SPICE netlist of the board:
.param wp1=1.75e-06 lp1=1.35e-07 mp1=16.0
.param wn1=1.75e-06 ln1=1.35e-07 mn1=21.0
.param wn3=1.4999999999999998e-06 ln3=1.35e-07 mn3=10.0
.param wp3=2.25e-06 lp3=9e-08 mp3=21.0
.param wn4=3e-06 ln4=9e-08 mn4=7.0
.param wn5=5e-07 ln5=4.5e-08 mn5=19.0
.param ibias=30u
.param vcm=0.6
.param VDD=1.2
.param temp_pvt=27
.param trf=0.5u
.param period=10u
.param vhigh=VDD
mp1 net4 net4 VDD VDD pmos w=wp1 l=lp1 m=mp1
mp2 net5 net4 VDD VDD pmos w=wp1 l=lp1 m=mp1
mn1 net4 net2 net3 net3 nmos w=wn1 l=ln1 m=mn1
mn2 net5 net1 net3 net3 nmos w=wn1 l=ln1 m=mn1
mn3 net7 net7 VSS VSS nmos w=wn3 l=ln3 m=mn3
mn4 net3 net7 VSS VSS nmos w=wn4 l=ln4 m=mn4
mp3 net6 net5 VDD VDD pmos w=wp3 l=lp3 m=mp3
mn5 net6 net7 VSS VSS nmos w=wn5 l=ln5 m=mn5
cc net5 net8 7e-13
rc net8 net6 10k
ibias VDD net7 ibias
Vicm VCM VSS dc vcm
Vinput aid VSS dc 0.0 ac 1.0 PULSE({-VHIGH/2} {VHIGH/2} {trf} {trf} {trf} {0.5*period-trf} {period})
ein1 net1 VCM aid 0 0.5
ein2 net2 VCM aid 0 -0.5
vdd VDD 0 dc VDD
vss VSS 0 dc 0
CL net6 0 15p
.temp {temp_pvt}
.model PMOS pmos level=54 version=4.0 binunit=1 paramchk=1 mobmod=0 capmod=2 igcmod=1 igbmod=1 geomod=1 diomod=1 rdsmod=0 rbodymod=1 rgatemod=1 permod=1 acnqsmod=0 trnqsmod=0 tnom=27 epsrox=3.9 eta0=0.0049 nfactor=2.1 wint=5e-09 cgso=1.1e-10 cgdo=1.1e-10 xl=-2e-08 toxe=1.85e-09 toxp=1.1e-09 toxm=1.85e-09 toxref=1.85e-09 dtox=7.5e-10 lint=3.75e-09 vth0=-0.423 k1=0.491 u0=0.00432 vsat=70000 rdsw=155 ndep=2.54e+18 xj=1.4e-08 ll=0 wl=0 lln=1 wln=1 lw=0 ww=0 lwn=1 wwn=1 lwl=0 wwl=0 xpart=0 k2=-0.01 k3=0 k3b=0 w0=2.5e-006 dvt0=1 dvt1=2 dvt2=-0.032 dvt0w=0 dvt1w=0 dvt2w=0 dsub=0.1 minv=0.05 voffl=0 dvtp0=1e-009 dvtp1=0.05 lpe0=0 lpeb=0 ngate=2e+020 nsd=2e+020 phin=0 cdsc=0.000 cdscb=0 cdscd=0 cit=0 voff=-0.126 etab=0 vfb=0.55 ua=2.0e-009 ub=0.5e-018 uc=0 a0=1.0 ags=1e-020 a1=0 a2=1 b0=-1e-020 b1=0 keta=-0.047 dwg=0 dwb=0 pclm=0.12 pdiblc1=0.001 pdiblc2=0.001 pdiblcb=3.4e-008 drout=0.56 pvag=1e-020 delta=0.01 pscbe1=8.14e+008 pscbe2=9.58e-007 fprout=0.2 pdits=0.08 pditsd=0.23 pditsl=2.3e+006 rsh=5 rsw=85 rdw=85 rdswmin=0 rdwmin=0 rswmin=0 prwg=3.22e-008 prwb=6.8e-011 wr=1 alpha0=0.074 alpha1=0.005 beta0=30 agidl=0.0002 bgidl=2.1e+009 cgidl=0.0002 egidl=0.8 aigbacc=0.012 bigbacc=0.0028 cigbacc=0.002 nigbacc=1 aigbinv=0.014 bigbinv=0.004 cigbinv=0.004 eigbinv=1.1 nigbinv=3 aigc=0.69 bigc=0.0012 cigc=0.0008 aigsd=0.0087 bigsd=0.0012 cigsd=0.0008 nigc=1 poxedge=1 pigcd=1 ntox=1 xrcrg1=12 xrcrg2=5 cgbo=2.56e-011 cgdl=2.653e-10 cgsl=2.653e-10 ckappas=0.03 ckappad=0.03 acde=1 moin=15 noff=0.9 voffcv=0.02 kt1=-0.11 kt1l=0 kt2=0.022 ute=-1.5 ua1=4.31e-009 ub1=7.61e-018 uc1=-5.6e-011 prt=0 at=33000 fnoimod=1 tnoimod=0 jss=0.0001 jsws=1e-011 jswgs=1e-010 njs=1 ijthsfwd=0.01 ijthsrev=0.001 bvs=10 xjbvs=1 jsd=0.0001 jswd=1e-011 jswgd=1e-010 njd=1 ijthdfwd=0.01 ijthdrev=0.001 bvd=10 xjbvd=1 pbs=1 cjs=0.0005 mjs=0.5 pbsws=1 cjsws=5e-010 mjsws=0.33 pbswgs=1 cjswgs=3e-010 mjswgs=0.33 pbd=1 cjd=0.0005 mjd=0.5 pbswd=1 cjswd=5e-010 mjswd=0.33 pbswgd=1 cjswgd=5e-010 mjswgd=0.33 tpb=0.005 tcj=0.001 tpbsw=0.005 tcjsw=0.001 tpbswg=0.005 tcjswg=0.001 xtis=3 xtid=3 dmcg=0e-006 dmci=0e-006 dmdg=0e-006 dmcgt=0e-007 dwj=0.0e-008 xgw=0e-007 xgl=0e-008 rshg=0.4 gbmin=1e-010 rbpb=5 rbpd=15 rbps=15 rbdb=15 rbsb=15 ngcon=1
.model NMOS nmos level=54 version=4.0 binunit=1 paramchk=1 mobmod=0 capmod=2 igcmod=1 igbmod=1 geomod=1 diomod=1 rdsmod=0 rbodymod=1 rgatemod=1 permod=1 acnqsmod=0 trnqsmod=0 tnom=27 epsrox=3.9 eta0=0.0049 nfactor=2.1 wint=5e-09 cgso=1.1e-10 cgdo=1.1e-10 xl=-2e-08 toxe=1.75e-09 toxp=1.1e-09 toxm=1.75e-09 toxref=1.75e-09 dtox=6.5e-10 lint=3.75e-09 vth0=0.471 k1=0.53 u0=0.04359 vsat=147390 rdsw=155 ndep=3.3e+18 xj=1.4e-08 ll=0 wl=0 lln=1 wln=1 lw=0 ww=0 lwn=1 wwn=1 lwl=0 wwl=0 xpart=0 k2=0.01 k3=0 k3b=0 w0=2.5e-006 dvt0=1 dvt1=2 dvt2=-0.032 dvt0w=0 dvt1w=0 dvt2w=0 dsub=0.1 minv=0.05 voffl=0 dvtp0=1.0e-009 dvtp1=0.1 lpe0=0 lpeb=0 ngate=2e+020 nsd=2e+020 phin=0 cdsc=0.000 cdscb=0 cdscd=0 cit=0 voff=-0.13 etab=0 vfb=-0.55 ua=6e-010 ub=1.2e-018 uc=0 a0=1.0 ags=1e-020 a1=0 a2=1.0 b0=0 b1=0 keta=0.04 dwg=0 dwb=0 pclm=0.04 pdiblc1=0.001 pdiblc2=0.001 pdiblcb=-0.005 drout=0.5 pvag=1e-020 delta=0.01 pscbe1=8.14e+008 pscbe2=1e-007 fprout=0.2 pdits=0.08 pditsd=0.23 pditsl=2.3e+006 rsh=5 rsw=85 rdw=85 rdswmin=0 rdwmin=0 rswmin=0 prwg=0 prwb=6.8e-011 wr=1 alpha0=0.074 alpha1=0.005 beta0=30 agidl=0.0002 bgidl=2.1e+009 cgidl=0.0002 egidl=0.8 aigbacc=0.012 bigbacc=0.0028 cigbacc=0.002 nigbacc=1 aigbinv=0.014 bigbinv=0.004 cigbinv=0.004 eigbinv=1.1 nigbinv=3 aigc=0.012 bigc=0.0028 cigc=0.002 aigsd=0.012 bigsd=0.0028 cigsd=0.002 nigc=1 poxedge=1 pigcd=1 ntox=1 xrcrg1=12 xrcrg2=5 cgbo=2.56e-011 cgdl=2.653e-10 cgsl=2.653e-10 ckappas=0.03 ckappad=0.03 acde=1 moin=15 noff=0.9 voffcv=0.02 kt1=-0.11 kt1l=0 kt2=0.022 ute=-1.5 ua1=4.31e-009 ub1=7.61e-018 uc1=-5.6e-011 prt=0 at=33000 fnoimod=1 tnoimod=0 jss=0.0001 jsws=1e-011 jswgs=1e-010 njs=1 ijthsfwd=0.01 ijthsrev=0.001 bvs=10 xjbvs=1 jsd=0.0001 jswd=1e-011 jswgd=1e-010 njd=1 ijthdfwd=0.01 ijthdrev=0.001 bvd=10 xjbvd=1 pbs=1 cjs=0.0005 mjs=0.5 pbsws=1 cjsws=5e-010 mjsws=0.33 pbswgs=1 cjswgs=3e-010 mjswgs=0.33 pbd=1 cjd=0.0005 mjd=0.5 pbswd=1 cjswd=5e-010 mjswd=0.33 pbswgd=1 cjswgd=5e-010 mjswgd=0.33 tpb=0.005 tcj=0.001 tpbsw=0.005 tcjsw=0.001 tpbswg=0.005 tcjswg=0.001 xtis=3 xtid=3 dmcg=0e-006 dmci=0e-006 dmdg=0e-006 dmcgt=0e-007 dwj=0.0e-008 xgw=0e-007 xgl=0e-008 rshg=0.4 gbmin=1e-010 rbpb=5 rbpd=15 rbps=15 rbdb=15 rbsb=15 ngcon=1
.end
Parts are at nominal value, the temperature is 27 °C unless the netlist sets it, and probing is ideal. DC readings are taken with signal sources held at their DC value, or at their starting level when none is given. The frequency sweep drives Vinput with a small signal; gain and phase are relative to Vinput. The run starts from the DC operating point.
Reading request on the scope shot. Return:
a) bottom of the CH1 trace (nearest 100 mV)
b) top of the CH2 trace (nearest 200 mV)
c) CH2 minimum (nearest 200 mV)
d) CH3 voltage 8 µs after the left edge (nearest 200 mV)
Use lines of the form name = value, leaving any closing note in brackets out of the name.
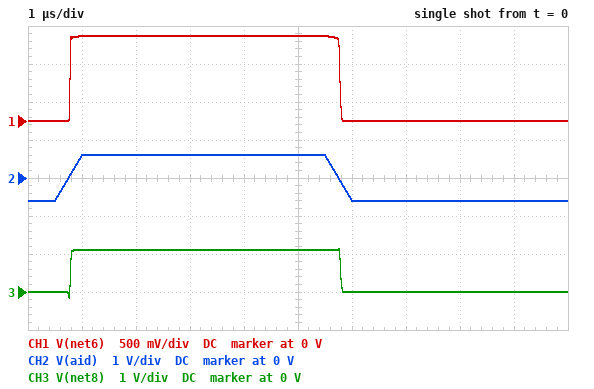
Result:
bottom of the CH1 trace = 0 V
top of the CH2 trace = 600 mV
CH2 minimum = -600 mV
CH3 voltage 8 µs after the left edge = 0 V
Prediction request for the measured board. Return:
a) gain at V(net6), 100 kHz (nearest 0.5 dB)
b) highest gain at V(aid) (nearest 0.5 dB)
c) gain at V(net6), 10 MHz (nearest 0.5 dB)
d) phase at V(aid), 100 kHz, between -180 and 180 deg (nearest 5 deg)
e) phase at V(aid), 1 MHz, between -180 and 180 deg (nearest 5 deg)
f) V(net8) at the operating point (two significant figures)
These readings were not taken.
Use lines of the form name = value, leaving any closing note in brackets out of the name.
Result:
gain at V(net6), 100 kHz = 47.5 dB
highest gain at V(aid) = 0 dB
gain at V(net6), 10 MHz = 21.5 dB
phase at V(aid), 100 kHz, between -180 and 180 deg = 0 deg
phase at V(aid), 1 MHz, between -180 and 180 deg = 0 deg
V(net8) at the operating point = 110 mV
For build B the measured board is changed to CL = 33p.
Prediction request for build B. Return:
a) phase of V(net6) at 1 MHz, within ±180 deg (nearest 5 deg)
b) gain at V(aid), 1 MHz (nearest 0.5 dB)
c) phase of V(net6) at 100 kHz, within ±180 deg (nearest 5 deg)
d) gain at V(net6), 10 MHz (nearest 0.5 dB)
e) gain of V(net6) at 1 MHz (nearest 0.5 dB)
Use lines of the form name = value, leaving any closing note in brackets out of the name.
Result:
phase of V(net6) at 1 MHz, within ±180 deg = -70 deg
gain at V(aid), 1 MHz = 0 dB
phase of V(net6) at 100 kHz, within ±180 deg = -15 deg
gain at V(net6), 10 MHz = 19.5 dB
gain of V(net6) at 1 MHz = 40.0 dB
